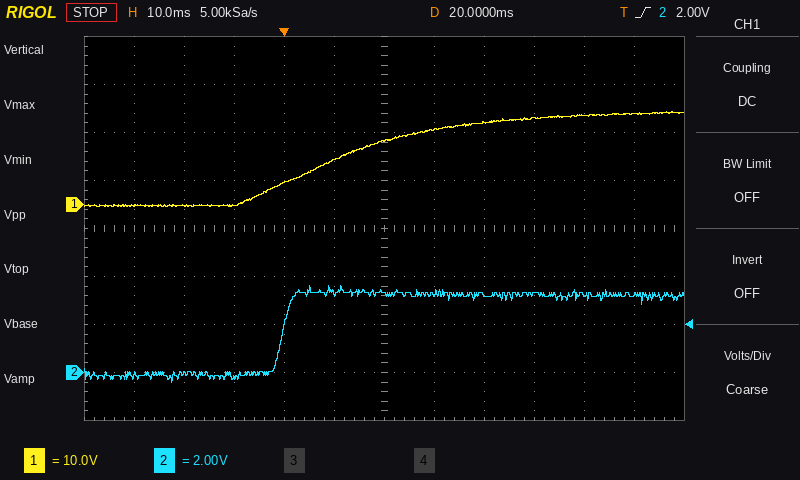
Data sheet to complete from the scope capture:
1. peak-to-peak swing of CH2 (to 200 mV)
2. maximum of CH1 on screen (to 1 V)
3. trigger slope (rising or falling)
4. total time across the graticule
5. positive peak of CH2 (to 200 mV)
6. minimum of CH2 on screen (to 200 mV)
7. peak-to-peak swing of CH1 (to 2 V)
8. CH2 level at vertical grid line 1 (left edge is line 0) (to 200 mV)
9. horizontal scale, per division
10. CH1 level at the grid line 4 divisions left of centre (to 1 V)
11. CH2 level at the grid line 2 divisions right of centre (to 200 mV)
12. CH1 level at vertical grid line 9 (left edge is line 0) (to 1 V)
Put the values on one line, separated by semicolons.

4.0 V; 19 V; rising; 120 ms; 3.6 V; -400 mV; 20 V; -200 mV; 10 ms; 0 V; 3.2 V; 18 V
